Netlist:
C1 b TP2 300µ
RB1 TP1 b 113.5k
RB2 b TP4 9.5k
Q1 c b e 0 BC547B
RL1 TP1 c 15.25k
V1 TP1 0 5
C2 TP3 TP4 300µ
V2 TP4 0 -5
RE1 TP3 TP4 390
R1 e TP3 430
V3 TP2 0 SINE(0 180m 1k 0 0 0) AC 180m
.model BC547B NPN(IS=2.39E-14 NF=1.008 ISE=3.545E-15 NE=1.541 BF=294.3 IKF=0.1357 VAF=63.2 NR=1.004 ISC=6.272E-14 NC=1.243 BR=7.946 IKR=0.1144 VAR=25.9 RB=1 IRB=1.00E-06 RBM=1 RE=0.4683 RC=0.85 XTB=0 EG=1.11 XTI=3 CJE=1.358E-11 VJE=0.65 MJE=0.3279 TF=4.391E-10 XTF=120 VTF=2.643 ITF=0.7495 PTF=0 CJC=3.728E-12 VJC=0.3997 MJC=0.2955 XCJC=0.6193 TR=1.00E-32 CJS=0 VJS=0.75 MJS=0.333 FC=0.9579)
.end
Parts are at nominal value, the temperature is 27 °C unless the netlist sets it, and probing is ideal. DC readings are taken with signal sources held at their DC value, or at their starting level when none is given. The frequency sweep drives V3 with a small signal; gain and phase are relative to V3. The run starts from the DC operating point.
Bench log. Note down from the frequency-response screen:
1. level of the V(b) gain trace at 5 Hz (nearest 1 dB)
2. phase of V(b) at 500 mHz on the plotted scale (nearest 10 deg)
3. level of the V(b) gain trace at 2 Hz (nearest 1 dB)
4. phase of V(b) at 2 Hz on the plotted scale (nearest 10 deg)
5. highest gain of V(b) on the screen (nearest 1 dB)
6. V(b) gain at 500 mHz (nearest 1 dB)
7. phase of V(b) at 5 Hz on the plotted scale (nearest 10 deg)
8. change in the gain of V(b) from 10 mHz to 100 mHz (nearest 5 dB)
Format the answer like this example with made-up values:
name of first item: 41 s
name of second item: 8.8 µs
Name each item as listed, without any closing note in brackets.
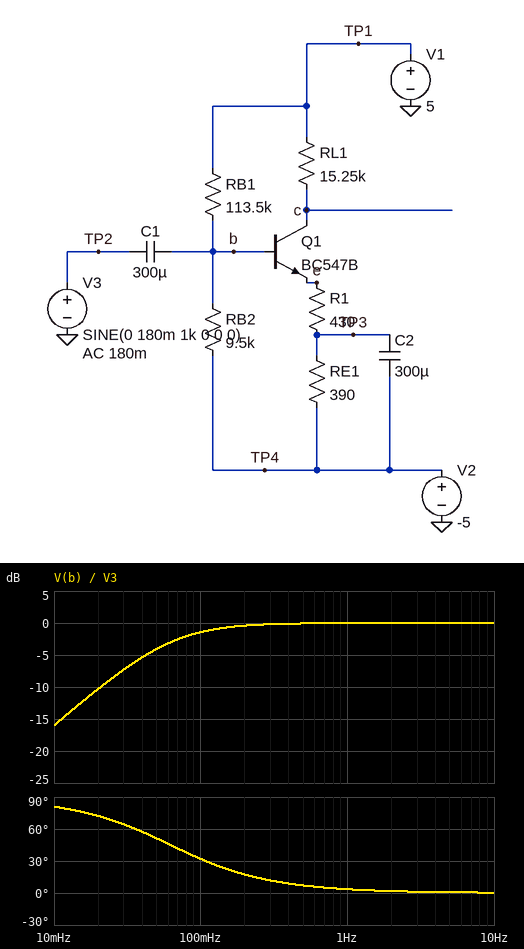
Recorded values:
level of the V(b) gain trace at 5 Hz: 0 dB
phase of V(b) at 500 mHz on the plotted scale: 10 deg
level of the V(b) gain trace at 2 Hz: 0 dB
phase of V(b) at 2 Hz on the plotted scale: 0 deg
highest gain of V(b) on the screen: 0 dB
V(b) gain at 500 mHz: 0 dB
phase of V(b) at 5 Hz on the plotted scale: 0 deg
change in the gain of V(b) from 10 mHz to 100 mHz: 15 dB
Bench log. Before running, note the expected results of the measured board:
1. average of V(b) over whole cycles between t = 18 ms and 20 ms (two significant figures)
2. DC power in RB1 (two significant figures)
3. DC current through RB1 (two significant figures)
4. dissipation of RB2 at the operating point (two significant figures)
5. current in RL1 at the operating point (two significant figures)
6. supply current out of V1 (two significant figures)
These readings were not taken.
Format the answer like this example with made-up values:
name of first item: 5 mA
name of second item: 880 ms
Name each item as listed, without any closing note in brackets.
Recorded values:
average of V(b) over whole cycles between t = 18 ms and 20 ms: -4.2 V
DC power in RB1: 750 µW
DC current through RB1: 81 µA
dissipation of RB2 at the operating point: 62 µW
current in RL1 at the operating point: 210 µA
supply current out of V1: 290 µA
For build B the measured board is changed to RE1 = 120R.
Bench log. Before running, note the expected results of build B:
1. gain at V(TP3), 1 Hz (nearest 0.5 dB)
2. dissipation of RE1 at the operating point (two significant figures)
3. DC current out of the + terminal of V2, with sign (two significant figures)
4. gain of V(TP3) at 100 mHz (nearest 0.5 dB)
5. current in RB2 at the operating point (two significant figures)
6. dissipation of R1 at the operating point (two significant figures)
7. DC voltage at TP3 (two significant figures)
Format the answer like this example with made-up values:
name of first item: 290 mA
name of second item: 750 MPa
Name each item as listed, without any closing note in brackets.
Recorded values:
gain at V(TP3), 1 Hz: -15.0 dB
dissipation of RE1 at the operating point: 10 µW
DC current out of the + terminal of V2, with sign: -370 µA
gain of V(TP3) at 100 mHz: -16.0 dB
current in RB2 at the operating point: 80 µA
dissipation of R1 at the operating point: 36 µW
DC voltage at TP3: -5.0 V
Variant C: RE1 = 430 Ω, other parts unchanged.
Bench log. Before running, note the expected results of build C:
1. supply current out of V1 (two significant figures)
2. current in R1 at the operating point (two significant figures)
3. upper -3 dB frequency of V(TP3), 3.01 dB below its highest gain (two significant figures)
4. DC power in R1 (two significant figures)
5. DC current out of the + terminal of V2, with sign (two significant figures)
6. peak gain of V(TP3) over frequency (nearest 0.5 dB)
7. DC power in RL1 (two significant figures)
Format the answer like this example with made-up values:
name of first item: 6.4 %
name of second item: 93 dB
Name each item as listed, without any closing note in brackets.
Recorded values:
supply current out of V1: 280 µA
current in R1 at the operating point: 200 µA
upper -3 dB frequency of V(TP3), 3.01 dB below its highest gain: 2.3 Hz
DC power in R1: 17 µW
DC current out of the + terminal of V2, with sign: -280 µA
peak gain of V(TP3) over frequency: -7.5 dB
DC power in RL1: 610 µW
